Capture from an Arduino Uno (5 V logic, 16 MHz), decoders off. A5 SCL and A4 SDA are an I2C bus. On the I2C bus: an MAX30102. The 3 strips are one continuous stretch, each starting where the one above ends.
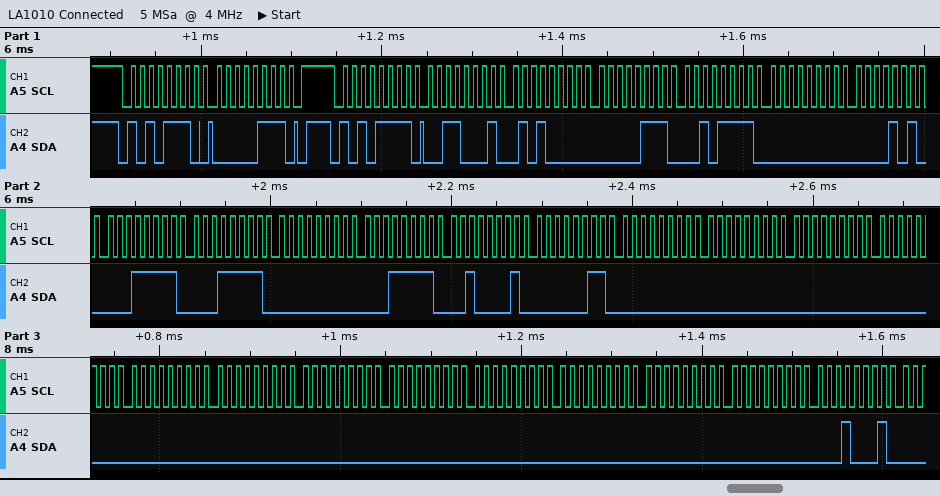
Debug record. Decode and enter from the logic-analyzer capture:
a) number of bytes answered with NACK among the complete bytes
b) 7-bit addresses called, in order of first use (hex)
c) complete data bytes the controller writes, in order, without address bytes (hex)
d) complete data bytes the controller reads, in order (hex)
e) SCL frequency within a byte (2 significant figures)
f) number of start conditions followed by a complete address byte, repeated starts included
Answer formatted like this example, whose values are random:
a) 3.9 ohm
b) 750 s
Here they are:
a) 0
b) 0x57
c) 07
d) 31 50 07 2F 00 0A 1F 1F 00 1F 21 03 00 00 00 00 00 00 00 00 00 00 00 00 11
e) 100 kHz
f) 2
